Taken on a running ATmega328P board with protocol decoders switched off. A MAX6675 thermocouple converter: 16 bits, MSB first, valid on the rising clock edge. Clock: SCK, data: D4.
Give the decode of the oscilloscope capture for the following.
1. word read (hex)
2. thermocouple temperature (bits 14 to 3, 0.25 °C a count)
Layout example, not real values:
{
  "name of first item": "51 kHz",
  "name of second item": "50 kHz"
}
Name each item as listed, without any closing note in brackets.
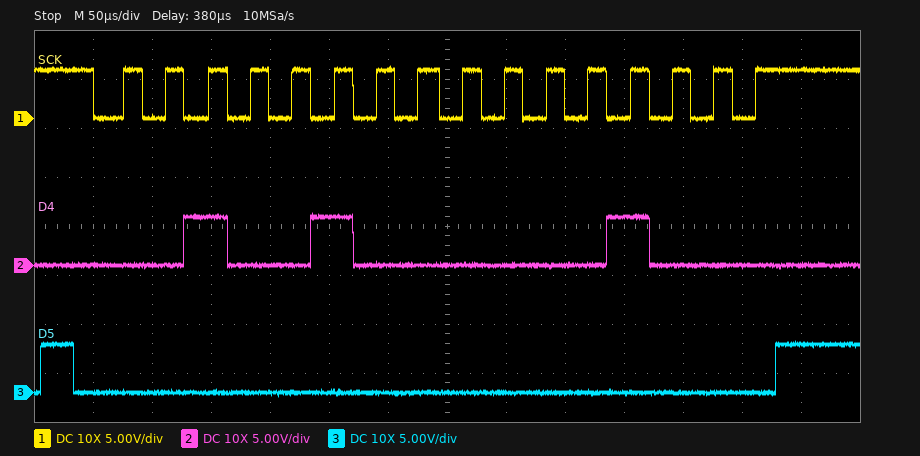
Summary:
{
  "word read": "0x2408",
  "thermocouple temperature": "288.25 °C"
}
